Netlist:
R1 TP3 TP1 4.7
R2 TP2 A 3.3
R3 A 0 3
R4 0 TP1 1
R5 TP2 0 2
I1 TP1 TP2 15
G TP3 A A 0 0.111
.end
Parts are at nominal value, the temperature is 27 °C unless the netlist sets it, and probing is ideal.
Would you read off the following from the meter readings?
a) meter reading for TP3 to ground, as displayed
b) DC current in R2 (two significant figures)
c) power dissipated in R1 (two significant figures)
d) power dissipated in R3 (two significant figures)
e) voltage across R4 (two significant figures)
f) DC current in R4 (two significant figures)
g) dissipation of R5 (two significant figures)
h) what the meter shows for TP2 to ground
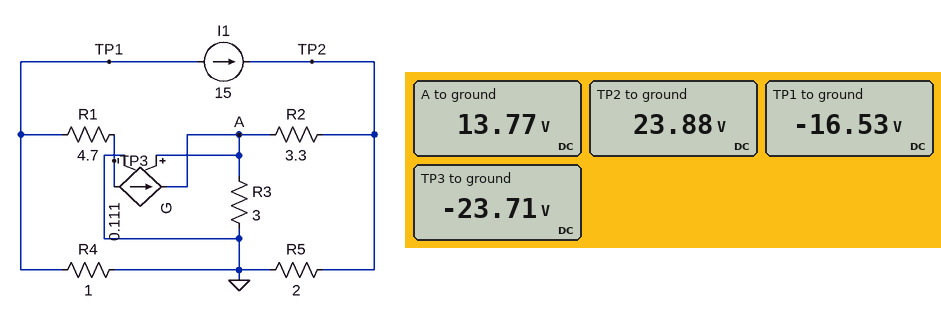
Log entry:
-23.71 V
3.1 A
11 W
63 W
17 V
17 A
290 W
23.88 V
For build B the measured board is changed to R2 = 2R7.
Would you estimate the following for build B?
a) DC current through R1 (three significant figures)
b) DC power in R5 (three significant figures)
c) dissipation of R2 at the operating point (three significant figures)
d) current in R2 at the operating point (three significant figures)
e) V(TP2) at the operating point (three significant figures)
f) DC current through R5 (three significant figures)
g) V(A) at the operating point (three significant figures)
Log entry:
1.63 A
276 W
28.7 W
3.26 A
23.5 V
11.7 A
14.7 V
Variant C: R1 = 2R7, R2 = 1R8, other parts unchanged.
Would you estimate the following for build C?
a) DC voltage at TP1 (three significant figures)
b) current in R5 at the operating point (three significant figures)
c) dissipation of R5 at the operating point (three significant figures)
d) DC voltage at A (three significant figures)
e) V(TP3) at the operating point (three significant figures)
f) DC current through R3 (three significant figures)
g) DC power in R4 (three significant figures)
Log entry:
-16.8 V
11.4 A
259 W
16.3 V
-21.7 V
5.42 A
282 W
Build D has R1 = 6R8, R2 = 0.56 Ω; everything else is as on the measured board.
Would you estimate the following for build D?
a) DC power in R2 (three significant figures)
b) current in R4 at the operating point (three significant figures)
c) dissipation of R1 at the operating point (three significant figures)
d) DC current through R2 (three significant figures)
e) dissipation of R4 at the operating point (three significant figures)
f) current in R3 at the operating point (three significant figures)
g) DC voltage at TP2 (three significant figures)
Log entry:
10.1 W
17.1 A
30.6 W
4.25 A
293 W
6.37 A
21.5 V
